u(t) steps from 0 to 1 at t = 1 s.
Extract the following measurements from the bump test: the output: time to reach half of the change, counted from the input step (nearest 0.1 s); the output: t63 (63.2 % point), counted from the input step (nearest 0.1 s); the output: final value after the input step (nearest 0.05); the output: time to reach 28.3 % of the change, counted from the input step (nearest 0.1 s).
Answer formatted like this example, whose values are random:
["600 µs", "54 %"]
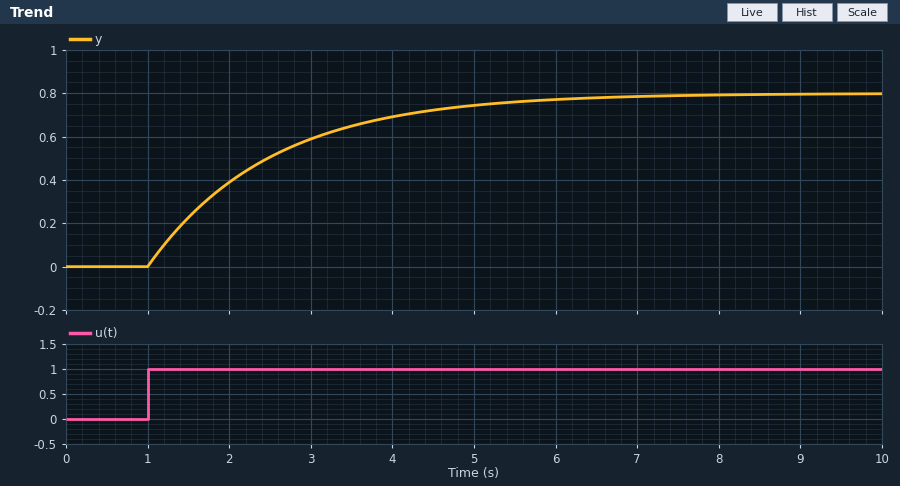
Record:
["1.0 s", "1.5 s", "0.80", "0.5 s"]
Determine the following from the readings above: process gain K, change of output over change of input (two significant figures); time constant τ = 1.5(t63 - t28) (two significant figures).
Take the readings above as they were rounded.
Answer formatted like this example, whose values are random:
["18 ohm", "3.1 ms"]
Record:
["0.80", "1.5 s"]
